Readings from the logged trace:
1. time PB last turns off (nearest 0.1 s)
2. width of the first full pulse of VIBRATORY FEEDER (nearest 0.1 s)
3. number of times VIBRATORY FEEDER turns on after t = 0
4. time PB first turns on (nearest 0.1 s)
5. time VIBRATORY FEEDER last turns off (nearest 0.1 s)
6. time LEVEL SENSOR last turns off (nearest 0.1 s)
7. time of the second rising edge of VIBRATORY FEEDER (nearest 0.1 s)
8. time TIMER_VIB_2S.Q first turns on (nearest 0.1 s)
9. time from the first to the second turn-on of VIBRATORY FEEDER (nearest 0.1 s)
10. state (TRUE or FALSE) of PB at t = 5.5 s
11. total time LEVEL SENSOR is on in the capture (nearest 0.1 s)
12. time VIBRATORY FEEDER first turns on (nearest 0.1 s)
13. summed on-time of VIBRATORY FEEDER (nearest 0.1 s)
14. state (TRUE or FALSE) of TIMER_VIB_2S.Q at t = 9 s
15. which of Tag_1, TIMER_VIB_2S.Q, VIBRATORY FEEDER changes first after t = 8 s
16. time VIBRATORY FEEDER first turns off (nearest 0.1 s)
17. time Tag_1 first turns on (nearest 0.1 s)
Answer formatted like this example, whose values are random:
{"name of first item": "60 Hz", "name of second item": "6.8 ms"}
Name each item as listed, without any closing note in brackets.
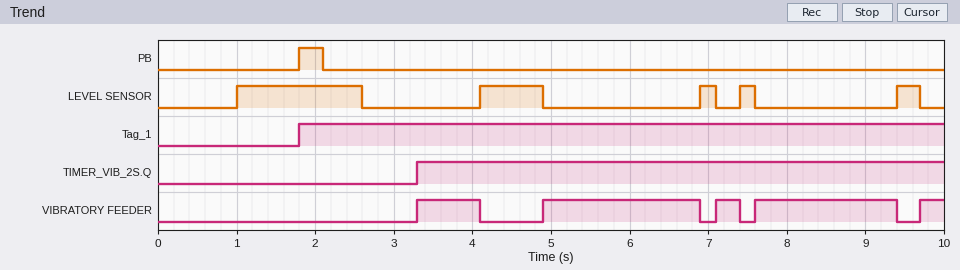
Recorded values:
{"time PB last turns off": "2.1 s", "width of the first full pulse of VIBRATORY FEEDER": "0.8 s", "number of times VIBRATORY FEEDER turns on after t = 0": "5", "time PB first turns on": "1.8 s", "time VIBRATORY FEEDER last turns off": "9.4 s", "time LEVEL SENSOR last turns off": "9.7 s", "time of the second rising edge of VIBRATORY FEEDER": "4.9 s", "time TIMER_VIB_2S.Q first turns on": "3.3 s", "time from the first to the second turn-on of VIBRATORY FEEDER": "1.6 s", "state (TRUE or FALSE) of PB at t = 5.5 s": "FALSE", "total time LEVEL SENSOR is on in the capture": "3.1 s", "time VIBRATORY FEEDER first turns on": "3.3 s", "summed on-time of VIBRATORY FEEDER": "5.2 s", "state (TRUE or FALSE) of TIMER_VIB_2S.Q at t = 9 s": "TRUE", "which of Tag_1, TIMER_VIB_2S.Q, VIBRATORY FEEDER changes first after t = 8 s": "VIBRATORY FEEDER", "time VIBRATORY FEEDER first turns off": "4.1 s", "time Tag_1 first turns on": "1.8 s"}
